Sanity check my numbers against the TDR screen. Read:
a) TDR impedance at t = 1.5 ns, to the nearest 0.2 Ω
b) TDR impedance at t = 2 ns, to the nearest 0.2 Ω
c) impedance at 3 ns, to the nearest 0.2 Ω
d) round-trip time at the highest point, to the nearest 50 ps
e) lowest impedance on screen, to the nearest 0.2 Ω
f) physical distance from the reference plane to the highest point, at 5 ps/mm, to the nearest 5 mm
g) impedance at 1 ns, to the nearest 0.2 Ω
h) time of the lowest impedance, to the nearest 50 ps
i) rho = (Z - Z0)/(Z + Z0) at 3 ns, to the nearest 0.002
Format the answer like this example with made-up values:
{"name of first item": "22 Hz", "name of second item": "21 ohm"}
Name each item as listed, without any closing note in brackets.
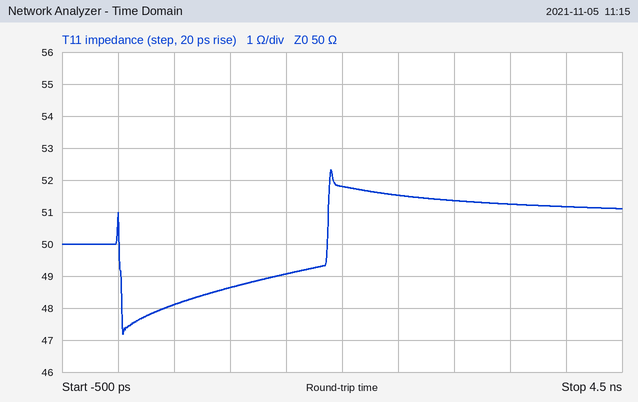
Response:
{"TDR impedance at t = 1.5 ns, to the nearest 0.2 Ω": "49.0 Ω", "TDR impedance at t = 2 ns, to the nearest 0.2 Ω": "51.8 Ω", "impedance at 3 ns, to the nearest 0.2 Ω": "51.4 Ω", "round-trip time at the highest point, to the nearest 50 ps": "1.90 ns", "lowest impedance on screen, to the nearest 0.2 Ω": "47.2 Ω", "physical distance from the reference plane to the highest point, at 5 ps/mm, to the nearest 5 mm": "190 mm", "impedance at 1 ns, to the nearest 0.2 Ω": "48.6 Ω", "time of the lowest impedance, to the nearest 50 ps": "50 ps", "rho = (Z - Z0)/(Z + Z0) at 3 ns, to the nearest 0.002": "+0.014"}
